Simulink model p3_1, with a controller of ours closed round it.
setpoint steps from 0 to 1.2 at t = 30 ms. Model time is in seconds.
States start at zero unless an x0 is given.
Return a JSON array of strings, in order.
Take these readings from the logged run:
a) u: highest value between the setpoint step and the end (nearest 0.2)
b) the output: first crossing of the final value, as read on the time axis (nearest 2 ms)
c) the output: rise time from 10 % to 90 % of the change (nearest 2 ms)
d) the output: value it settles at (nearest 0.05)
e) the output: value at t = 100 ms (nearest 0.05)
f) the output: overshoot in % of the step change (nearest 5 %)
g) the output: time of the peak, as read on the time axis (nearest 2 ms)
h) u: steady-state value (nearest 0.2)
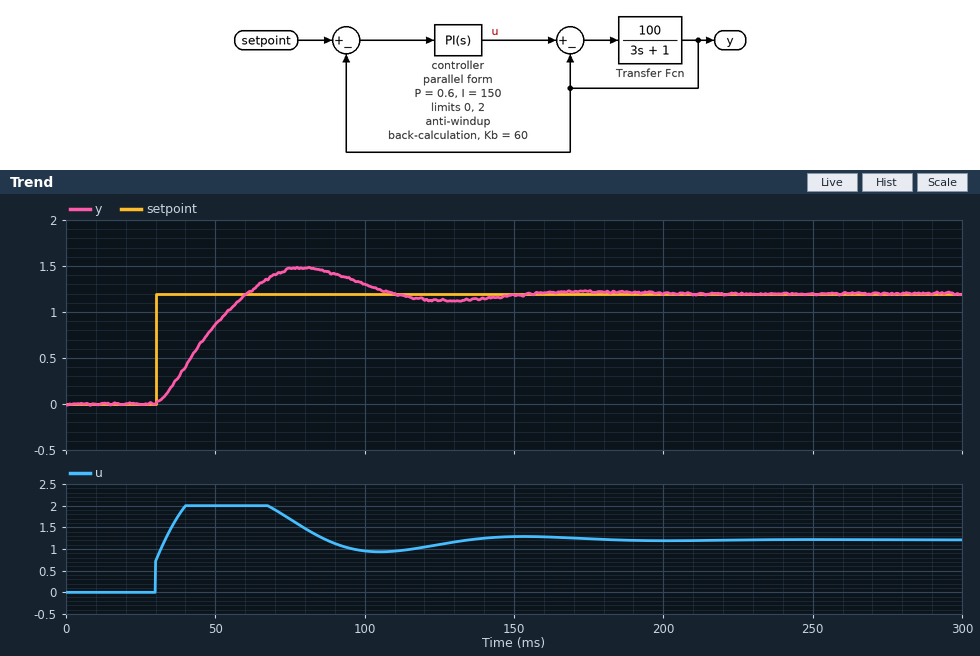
["2.0", "60 ms", "22 ms", "1.20", "1.30", "25 %", "80 ms", "1.2"]
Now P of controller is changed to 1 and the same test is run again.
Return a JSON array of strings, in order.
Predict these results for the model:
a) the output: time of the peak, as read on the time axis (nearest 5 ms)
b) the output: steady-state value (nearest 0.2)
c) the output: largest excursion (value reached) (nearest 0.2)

["75 ms", "1.2", "1.4"]
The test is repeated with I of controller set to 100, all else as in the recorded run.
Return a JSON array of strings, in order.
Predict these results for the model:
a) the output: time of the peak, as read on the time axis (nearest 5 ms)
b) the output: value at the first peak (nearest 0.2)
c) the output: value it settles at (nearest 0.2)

["85 ms", "1.4", "1.2"]
